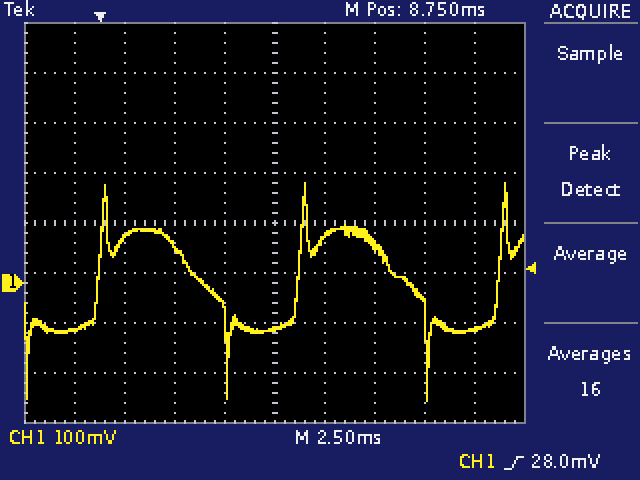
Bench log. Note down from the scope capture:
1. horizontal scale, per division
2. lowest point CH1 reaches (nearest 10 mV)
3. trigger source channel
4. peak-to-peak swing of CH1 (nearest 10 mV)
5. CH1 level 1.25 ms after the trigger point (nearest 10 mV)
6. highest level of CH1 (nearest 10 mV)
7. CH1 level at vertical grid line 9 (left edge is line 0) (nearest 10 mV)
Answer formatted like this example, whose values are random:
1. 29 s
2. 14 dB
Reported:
1. 2.5 ms
2. -240 mV
3. CH1
4. 440 mV
5. 90 mV
6. 200 mV
7. -90 mV
